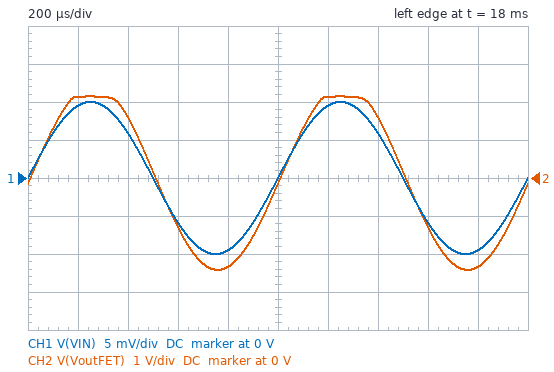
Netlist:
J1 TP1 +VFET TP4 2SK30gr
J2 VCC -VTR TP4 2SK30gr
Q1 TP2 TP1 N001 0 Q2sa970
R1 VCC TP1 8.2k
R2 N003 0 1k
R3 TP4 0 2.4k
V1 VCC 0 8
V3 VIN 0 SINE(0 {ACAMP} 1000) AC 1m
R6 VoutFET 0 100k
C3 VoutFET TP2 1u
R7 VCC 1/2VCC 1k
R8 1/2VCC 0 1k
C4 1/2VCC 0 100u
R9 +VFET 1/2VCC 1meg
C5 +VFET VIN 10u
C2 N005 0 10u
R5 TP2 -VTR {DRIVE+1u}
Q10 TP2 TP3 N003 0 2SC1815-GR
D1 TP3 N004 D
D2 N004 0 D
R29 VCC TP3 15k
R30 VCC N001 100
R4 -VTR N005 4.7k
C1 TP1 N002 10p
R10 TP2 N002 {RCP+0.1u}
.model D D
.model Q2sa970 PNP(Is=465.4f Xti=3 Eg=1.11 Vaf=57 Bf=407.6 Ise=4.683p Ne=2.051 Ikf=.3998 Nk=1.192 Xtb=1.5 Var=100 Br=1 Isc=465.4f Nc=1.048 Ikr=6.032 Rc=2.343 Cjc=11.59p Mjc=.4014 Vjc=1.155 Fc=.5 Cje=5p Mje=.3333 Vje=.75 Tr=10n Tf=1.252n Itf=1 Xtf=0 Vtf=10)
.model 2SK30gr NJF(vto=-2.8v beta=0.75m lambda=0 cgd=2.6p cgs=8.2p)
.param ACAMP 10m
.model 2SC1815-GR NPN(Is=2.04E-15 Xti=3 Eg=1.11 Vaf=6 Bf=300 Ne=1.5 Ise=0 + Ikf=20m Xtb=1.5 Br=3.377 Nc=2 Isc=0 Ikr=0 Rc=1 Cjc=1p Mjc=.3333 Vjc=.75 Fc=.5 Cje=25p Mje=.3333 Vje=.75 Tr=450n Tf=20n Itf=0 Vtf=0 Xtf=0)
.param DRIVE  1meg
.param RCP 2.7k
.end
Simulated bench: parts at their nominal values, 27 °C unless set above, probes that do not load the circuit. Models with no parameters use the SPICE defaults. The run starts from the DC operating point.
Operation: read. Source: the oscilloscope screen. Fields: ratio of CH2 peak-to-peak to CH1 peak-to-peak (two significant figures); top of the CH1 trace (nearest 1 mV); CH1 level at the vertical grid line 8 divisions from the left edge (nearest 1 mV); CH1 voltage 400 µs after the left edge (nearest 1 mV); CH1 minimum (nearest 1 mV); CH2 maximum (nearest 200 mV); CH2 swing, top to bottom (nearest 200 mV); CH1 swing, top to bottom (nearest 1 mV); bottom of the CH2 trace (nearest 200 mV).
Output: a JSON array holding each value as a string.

["230", "10 mV", "-6 mV", "6 mV", "-10 mV", "2.2 V", "4.6 V", "20 mV", "-2.4 V"]
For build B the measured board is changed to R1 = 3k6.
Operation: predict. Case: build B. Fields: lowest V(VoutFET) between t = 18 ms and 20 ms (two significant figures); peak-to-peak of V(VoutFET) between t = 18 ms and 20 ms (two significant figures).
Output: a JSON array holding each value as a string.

["-2.0 V", "4.0 V"]
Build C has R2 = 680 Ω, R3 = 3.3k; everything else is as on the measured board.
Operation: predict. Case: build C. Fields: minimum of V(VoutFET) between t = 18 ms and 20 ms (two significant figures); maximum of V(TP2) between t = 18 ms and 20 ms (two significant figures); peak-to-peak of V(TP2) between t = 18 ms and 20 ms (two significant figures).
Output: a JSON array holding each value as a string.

["-2.0 V", "7.3 V", "4.1 V"]
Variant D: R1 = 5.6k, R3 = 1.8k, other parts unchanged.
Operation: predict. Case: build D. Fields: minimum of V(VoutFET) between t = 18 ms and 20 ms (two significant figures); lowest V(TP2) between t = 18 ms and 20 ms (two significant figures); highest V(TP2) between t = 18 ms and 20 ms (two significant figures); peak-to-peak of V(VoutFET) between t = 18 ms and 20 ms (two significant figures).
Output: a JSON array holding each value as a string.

["-2.6 V", "3.3 V", "7.8 V", "4.5 V"]
